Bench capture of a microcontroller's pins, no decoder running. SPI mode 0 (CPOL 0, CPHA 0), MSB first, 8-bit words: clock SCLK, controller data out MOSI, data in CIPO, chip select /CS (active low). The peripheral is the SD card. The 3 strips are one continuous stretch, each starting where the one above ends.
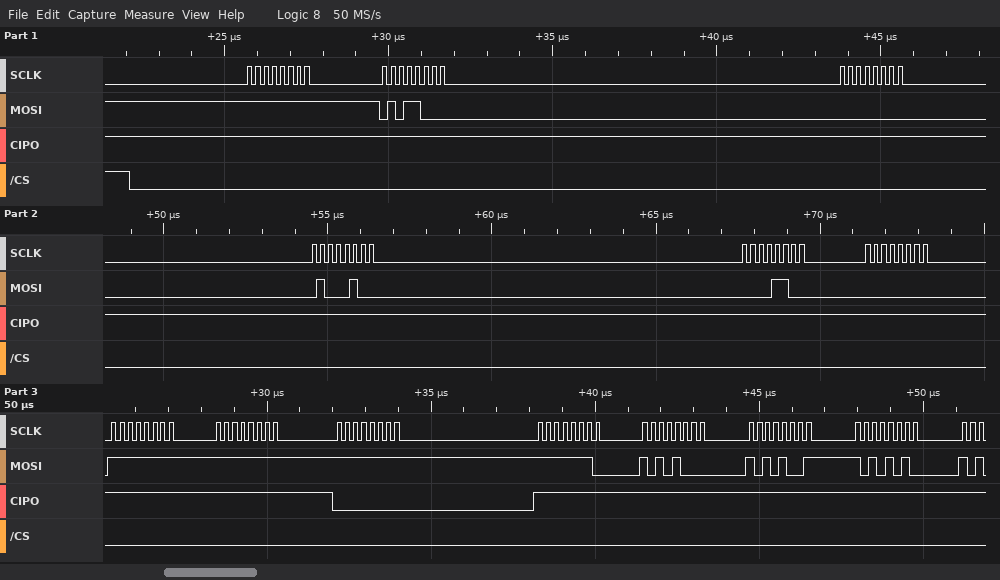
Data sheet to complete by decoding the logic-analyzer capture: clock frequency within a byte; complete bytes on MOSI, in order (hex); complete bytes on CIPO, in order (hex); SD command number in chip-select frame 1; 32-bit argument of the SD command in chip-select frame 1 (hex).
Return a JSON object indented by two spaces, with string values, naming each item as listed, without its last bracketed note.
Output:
{
  "clock frequency within a byte": "4 MHz",
  "complete bytes on MOSI, in order": "0xFF 0x58 0x00 0x44 0x0C 0x00 0xFF 0xFF 0xFF 0xFE 0xA8 0xA9 0xAA",
  "complete bytes on CIPO, in order": "0xFF 0xFF 0xFF 0xFF 0xFF 0xFF 0xFF 0xFF 0x00 0xFF 0xFF 0xFF 0xFF",
  "SD command number in chip-select frame 1": "CMD24",
  "32-bit argument of the SD command in chip-select frame 1": "0x00440C00"
}
